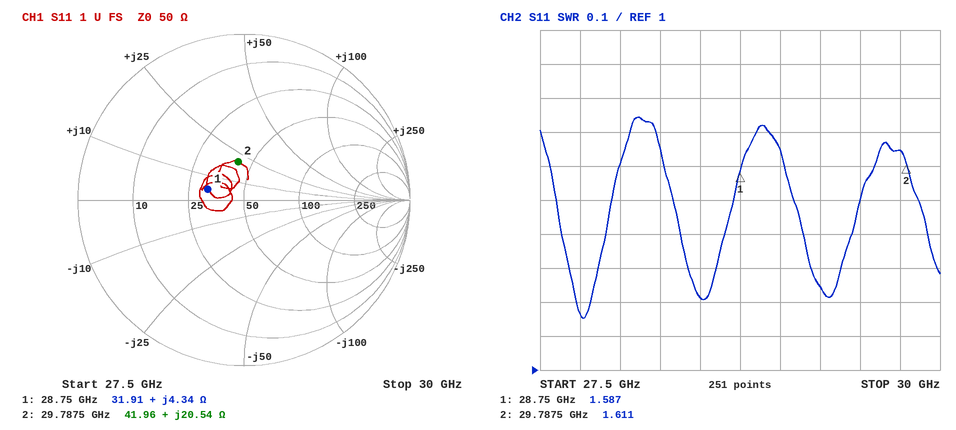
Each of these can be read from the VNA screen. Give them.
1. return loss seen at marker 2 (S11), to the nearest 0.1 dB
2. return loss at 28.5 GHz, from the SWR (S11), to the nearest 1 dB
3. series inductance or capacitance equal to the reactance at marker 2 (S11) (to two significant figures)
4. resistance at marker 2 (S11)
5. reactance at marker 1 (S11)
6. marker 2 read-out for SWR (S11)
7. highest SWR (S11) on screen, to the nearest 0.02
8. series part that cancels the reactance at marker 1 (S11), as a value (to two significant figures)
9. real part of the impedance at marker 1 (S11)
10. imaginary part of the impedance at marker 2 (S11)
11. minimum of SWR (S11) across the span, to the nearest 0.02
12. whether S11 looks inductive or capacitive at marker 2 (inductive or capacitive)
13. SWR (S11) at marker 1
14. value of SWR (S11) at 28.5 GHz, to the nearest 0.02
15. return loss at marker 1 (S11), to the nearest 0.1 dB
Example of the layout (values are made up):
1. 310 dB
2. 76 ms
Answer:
1. 12.6 dB
2. 20 dB
3. 110 pH
4. 41.96 Ω
5. +4.34 Ω
6. 1.611
7. 1.74
8. 1.3 pF
9. 31.91 Ω
10. +20.54 Ω
11. 1.16
12. inductive
13. 1.587
14. 1.22
15. 12.9 dB
